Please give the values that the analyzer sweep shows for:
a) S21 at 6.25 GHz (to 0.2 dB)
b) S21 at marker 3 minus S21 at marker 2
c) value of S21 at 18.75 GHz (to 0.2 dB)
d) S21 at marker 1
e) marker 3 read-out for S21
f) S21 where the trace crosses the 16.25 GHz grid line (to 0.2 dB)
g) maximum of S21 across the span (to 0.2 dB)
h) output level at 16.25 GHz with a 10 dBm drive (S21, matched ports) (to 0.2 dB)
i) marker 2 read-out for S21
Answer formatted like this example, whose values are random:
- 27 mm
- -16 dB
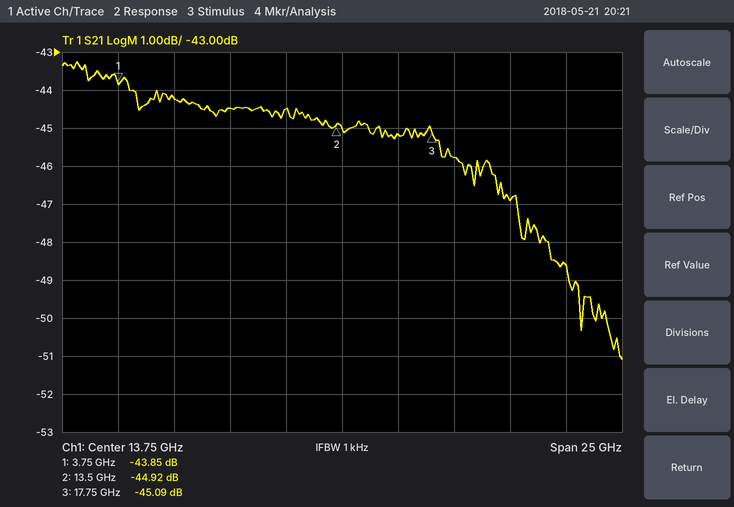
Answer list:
- -44.2 dB
- -0.17 dB
- -45.8 dB
- -43.85 dB
- -45.09 dB
- -45.2 dB
- -43.2 dB
- -35.2 dBm
- -44.92 dB
